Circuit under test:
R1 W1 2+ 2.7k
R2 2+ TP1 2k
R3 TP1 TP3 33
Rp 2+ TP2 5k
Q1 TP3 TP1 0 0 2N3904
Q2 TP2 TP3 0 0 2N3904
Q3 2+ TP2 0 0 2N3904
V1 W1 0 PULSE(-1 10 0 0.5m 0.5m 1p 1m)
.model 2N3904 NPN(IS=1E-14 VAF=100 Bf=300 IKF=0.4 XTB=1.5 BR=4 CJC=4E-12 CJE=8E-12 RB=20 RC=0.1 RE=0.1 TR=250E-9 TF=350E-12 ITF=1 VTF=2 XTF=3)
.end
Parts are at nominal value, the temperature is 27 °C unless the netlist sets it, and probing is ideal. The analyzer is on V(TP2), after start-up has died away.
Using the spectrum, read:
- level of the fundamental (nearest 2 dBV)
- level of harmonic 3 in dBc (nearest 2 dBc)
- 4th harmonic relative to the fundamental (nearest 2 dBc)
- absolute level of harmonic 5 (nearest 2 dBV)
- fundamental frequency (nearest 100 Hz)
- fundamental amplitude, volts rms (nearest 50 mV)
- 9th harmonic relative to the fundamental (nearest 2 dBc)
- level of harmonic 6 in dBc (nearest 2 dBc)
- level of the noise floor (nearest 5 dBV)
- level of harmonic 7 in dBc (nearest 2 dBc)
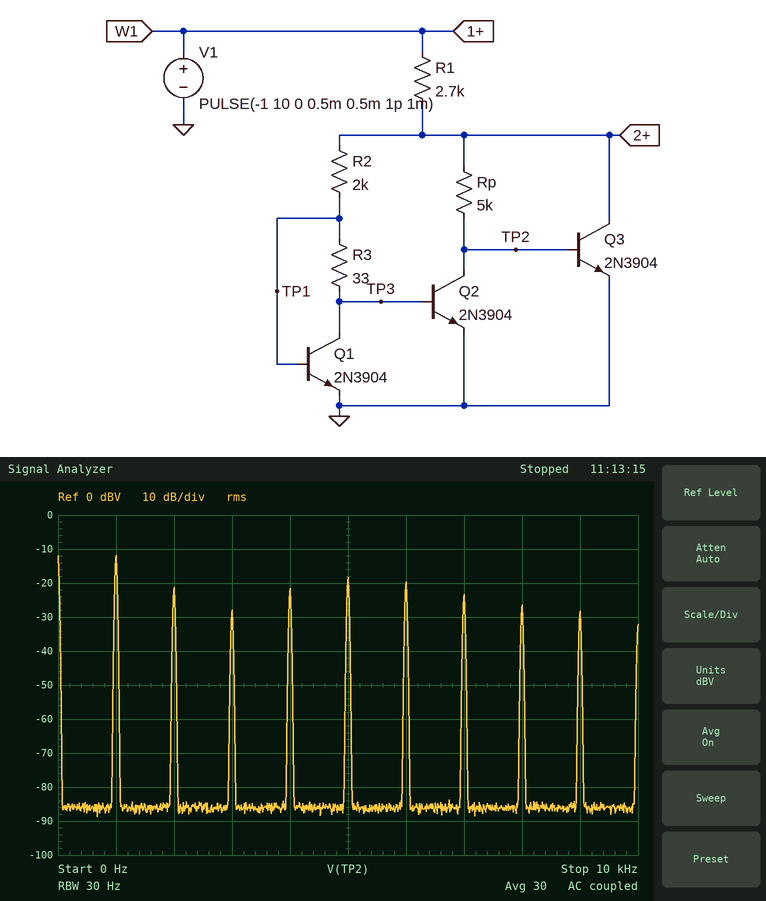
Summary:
-12 dBV
-16 dBc
-10 dBc
-18 dBV
1.0 kHz
250 mV
-16 dBc
-8 dBc
-85 dBV
-12 dBc
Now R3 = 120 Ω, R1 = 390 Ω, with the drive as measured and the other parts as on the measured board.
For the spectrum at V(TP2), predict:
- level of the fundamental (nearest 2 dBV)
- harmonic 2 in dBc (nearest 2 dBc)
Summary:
-14 dBV
-2 dBc
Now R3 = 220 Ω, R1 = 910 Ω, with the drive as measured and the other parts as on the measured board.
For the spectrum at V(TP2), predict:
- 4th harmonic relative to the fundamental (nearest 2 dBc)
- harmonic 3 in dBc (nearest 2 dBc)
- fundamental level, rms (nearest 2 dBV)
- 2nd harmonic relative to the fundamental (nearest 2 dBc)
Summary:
-4 dBc
-2 dBc
-14 dBV
-2 dBc
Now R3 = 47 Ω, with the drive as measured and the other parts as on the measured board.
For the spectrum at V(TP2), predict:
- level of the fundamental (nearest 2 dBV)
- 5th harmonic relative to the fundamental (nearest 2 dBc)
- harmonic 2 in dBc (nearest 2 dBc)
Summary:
-12 dBV
-8 dBc
-4 dBc
